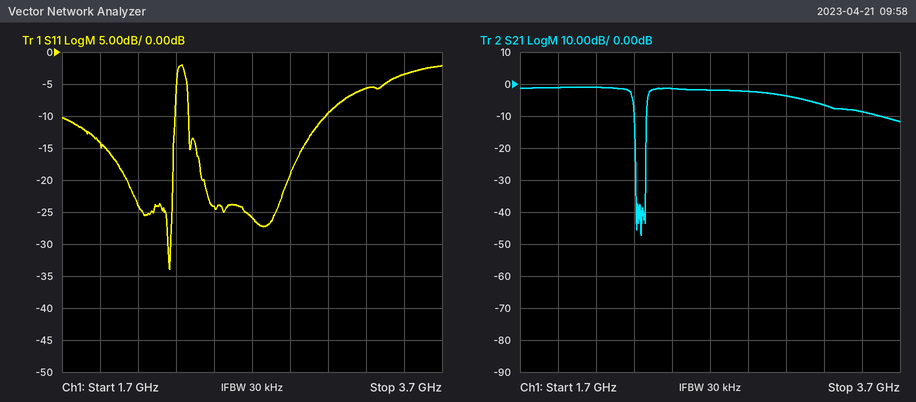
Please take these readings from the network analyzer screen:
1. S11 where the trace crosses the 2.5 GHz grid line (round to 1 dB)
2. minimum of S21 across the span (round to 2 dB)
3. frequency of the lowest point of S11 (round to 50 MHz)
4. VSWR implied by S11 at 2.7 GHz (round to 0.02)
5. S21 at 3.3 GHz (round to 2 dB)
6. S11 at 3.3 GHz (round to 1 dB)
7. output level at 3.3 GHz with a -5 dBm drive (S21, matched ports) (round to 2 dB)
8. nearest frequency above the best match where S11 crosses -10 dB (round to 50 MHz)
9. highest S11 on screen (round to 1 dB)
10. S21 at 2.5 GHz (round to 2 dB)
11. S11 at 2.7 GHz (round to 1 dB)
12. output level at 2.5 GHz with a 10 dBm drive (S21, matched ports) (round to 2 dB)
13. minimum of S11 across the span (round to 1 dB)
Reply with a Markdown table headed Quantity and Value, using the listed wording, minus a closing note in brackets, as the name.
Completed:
| Quantity | Value |
|---|---|
| S11 where the trace crosses the 2.5 GHz grid line | -24 dB |
| minimum of S21 across the span | -48 dB |
| frequency of the lowest point of S11 | 2.25 GHz |
| VSWR implied by S11 at 2.7 GHz | 1.10 |
| S21 at 3.3 GHz | -6 dB |
| S11 at 3.3 GHz | -6 dB |
| output level at 3.3 GHz with a -5 dBm drive (S21, matched ports) | -12 dBm |
| nearest frequency above the best match where S11 crosses -10 dB | 2.30 GHz |
| highest S11 on screen | -2 dB |
| S21 at 2.5 GHz | -2 dB |
| S11 at 2.7 GHz | -26 dB |
| output level at 2.5 GHz with a 10 dBm drive (S21, matched ports) | 8 dBm |
| minimum of S11 across the span | -34 dB |
